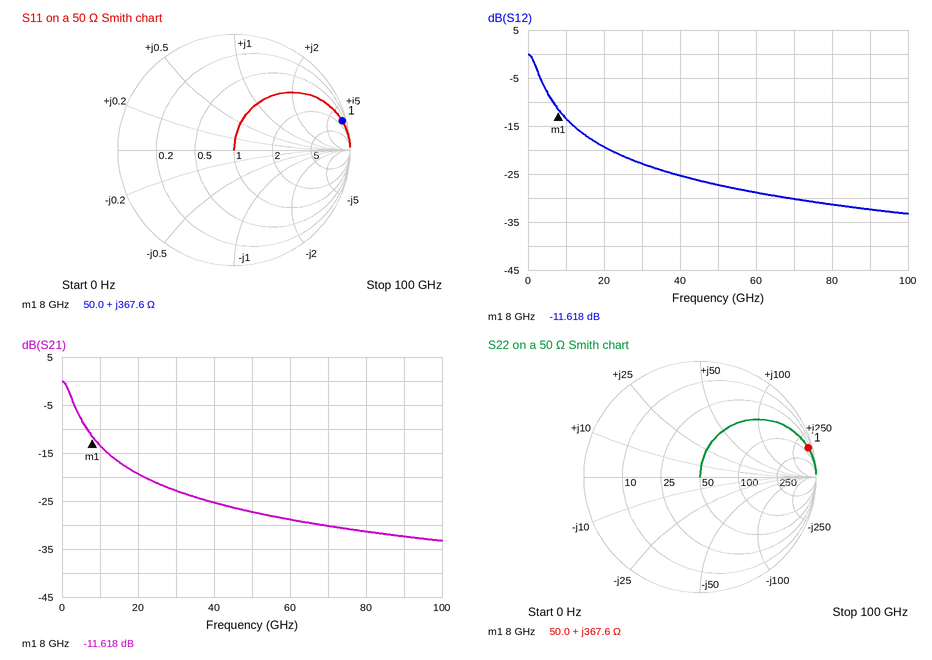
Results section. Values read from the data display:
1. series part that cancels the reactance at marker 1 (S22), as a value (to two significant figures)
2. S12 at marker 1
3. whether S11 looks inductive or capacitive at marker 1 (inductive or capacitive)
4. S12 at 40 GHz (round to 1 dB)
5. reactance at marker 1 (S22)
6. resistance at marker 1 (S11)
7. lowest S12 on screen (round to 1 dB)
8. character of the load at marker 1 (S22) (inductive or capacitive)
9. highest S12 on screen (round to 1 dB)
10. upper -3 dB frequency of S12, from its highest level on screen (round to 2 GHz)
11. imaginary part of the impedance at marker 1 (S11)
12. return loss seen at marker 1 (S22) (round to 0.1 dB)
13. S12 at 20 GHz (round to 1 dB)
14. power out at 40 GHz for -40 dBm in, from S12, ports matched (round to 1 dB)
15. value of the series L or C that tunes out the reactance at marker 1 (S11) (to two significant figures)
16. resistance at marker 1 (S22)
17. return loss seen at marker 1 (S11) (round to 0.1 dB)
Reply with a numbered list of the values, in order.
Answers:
1. 54 fF
2. -11.618 dB
3. inductive
4. -25 dB
5. +367.6 Ω
6. 50.0 Ω
7. -33 dB
8. inductive
9. 0 dB
10. 2 GHz
11. +367.6 Ω
12. 0.3 dB
13. -19 dB
14. -65 dBm
15. 54 fF
16. 50.0 Ω
17. 0.3 dB
